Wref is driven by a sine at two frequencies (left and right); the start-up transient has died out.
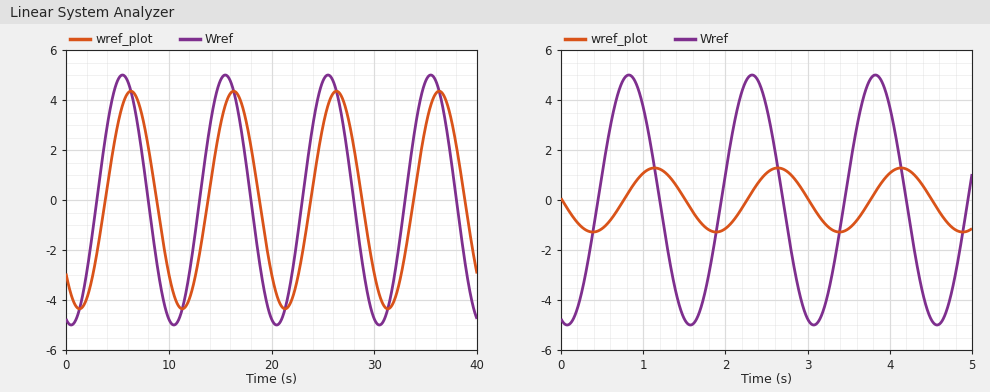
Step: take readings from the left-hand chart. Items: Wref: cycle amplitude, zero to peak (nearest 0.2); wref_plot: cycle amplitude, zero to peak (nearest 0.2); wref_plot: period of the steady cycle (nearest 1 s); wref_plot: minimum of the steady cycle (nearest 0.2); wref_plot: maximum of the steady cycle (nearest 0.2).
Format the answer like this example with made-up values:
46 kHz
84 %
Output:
5.0
4.4
10 s
-4.4
4.4
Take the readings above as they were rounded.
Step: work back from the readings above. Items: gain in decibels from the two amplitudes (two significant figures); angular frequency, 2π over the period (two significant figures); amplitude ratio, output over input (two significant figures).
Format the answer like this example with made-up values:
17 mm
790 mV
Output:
-1.1 dB
0.63 rad/s
0.88
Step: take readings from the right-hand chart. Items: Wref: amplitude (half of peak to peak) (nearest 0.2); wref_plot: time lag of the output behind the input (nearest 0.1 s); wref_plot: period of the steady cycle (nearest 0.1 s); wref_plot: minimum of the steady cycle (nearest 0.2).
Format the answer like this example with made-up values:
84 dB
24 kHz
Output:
5.0
0.3 s
1.5 s
-1.2
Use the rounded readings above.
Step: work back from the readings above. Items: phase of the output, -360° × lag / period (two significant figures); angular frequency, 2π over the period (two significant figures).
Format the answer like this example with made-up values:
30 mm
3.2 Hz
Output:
-72°
4.2 rad/s
